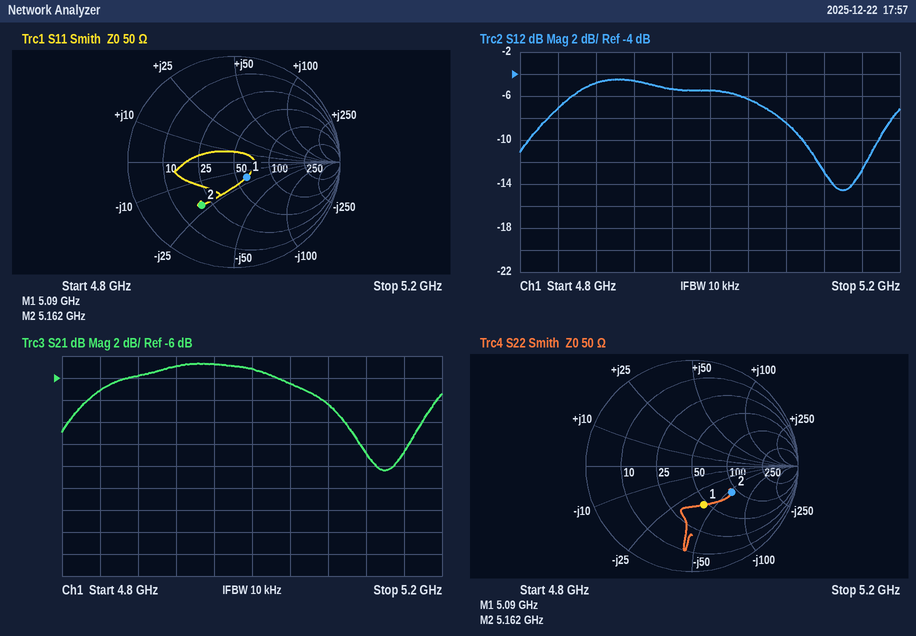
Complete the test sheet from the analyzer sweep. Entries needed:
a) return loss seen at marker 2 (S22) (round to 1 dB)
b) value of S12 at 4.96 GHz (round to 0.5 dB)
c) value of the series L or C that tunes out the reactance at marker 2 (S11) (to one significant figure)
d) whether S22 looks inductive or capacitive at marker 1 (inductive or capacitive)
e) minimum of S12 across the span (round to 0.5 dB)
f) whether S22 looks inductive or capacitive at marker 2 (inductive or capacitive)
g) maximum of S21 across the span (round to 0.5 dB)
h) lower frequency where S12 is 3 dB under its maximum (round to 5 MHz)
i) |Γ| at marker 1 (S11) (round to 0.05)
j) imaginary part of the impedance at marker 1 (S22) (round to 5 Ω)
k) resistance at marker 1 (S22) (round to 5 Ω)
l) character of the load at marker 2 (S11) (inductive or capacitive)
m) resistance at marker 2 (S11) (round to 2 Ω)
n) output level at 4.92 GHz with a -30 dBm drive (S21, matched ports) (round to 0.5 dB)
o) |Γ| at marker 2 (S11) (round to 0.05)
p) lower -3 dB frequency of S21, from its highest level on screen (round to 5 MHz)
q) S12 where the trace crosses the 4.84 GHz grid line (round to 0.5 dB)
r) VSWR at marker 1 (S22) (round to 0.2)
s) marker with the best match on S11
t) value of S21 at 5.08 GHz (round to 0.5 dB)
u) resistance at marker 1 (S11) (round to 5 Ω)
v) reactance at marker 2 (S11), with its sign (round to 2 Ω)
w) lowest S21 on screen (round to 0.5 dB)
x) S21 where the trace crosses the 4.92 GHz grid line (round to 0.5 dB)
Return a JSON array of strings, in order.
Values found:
["7 dB", "-5.5 dB", "700 pH", "capacitive", "-14.5 dB", "capacitive", "-4.5 dB", "4.835 GHz", "0.20", "-40 Ω", "45 Ω", "capacitive", "20 Ω", "-35.0 dBm", "0.50", "4.830 GHz", "-7.0 dB", "2.2", "marker 1", "-8.5 dB", "60 Ω", "-22 Ω", "-14.5 dB", "-5.0 dB"]
